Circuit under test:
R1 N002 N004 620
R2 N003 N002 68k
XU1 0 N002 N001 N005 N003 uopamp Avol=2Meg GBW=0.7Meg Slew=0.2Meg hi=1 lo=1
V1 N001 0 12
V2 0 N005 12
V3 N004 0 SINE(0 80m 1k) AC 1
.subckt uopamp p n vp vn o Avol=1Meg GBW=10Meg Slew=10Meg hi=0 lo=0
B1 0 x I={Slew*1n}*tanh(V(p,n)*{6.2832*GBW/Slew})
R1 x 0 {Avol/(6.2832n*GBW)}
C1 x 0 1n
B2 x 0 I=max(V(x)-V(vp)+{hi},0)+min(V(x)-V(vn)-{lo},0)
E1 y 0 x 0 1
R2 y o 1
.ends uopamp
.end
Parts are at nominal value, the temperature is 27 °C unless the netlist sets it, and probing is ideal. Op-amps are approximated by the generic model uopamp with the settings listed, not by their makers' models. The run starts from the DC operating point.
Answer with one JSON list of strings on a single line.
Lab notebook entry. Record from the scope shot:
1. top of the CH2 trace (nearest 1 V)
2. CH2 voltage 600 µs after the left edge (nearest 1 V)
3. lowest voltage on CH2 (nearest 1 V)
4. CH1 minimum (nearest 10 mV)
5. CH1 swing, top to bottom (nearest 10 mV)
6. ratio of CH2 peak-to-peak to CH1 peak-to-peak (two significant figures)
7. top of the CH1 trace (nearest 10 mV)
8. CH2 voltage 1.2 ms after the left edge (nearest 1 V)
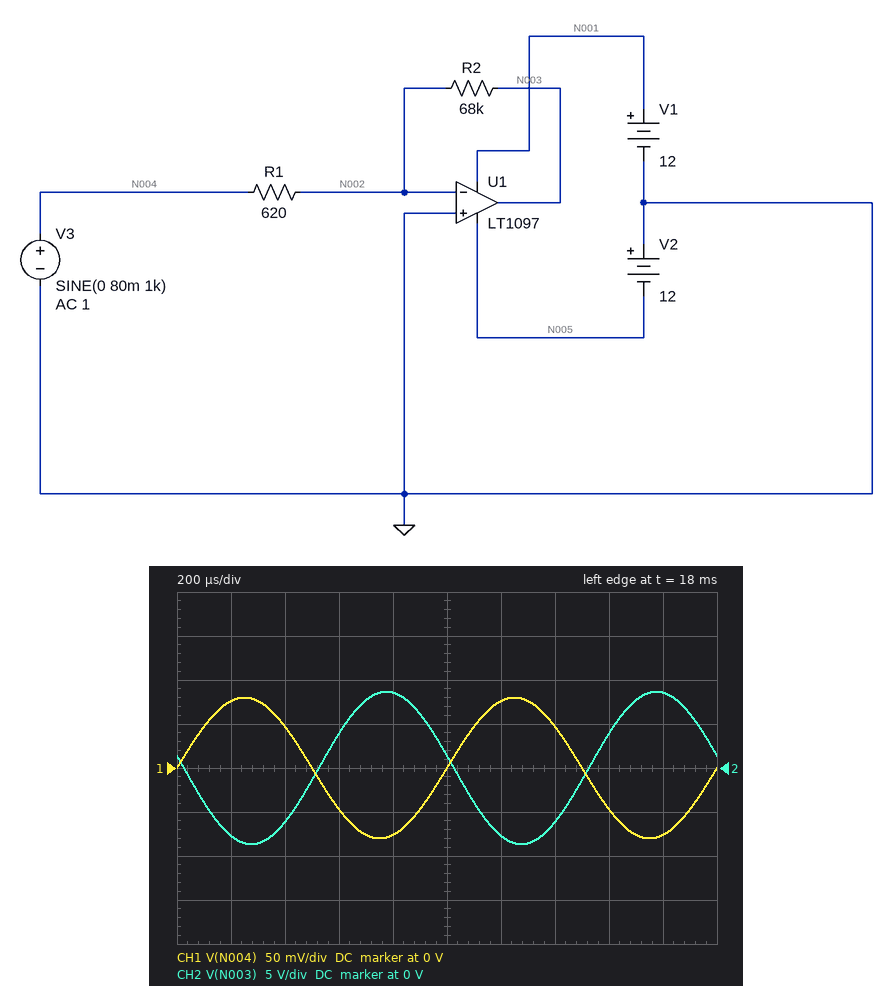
["9 V", "4 V", "-9 V", "-80 mV", "160 mV", "110", "80 mV", "-8 V"]
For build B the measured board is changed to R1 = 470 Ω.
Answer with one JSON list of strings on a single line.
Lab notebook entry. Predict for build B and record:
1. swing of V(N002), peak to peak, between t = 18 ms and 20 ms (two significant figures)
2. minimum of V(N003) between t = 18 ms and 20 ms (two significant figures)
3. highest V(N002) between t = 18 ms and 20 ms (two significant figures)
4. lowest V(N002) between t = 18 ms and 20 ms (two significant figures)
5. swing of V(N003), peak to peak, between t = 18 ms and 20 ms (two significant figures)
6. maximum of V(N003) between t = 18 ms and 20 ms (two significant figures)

["34 mV", "-11 V", "17 mV", "-17 mV", "22 V", "11 V"]
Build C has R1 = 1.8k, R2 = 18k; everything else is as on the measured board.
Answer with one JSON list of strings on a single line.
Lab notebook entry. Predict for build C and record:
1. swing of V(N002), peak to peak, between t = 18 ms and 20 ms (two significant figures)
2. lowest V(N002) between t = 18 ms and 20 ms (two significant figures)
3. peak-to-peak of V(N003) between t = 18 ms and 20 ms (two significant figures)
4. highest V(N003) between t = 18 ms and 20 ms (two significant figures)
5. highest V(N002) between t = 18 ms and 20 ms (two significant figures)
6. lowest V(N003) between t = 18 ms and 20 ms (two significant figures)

["2.3 mV", "-1.1 mV", "1.6 V", "800 mV", "1.1 mV", "-800 mV"]
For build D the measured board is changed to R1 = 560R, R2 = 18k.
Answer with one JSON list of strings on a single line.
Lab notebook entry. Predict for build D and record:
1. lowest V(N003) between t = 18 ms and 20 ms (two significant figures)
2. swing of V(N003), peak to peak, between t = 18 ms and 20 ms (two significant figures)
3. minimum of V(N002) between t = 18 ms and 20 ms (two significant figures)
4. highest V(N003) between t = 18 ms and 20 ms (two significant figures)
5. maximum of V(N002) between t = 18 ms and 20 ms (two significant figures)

["-2.6 V", "5.1 V", "-3.7 mV", "2.6 V", "3.7 mV"]
